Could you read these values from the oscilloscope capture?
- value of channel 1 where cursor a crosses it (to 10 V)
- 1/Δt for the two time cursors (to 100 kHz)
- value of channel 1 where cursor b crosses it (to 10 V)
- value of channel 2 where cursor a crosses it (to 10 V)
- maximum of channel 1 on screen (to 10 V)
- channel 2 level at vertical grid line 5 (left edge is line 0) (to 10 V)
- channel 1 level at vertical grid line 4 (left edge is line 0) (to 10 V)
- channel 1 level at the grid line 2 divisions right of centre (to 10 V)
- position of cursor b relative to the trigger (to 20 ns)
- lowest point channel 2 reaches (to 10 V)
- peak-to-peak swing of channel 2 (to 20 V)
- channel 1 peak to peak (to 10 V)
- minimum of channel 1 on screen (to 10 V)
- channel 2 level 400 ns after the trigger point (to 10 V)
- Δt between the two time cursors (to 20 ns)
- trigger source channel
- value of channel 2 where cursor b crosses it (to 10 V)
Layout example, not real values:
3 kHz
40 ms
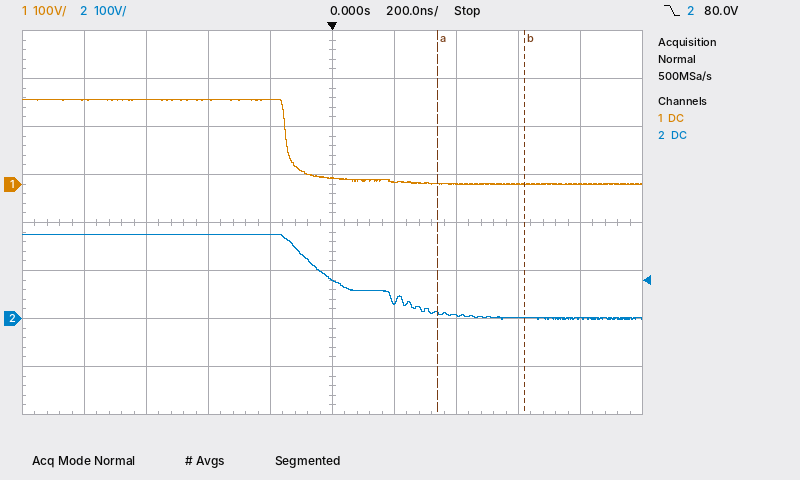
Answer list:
0 V
3.6 MHz
0 V
10 V
180 V
80 V
180 V
0 V
+620 ns
0 V
180 V
180 V
0 V
10 V
280 ns
channel 2
0 V
